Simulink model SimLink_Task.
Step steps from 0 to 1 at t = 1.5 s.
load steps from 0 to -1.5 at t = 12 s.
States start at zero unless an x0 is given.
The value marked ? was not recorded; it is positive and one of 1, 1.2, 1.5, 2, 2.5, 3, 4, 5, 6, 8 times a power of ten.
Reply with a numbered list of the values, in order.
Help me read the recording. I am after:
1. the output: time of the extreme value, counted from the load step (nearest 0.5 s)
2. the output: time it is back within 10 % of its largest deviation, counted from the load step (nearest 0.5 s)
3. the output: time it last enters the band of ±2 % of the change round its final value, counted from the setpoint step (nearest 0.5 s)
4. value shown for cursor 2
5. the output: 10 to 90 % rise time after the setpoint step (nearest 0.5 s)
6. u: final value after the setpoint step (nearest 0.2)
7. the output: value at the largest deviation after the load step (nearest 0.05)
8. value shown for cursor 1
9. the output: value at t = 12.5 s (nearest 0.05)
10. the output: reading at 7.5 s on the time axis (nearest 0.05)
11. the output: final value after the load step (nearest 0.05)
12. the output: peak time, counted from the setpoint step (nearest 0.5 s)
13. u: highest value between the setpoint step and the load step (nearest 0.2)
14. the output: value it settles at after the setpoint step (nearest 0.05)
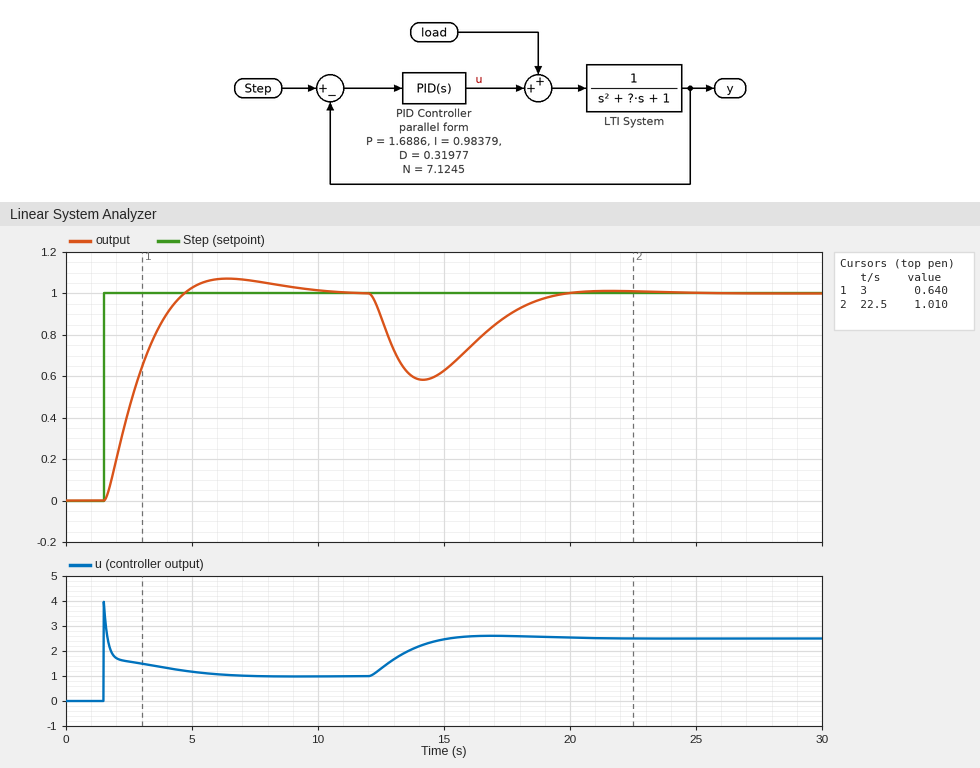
1. 2.0 s
2. 6.5 s
3. 8.0 s
4. 1.010
5. 2.0 s
6. 1.0
7. 0.60
8. 0.640
9. 0.90
10. 1.05
11. 1.00
12. 5.0 s
13. 4.0
14. 1.00
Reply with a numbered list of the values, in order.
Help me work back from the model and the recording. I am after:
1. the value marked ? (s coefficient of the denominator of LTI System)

1. 3
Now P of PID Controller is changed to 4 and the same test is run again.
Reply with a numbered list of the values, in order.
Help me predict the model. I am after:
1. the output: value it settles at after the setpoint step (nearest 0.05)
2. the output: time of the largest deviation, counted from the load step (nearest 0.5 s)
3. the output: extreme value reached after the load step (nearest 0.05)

1. 1.00
2. 1.5 s
3. 0.70
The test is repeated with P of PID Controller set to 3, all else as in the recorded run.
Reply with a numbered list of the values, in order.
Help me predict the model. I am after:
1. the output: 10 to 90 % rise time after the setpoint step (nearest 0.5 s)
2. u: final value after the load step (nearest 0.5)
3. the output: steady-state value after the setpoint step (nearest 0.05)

1. 1.5 s
2. 2.5
3. 1.00
